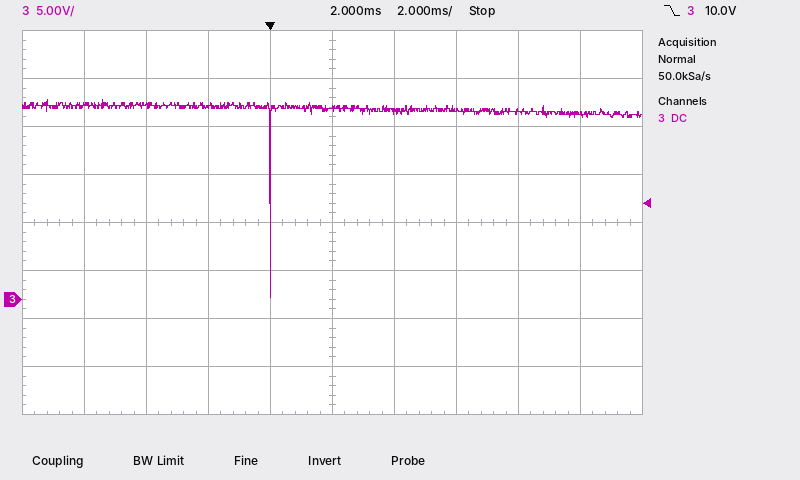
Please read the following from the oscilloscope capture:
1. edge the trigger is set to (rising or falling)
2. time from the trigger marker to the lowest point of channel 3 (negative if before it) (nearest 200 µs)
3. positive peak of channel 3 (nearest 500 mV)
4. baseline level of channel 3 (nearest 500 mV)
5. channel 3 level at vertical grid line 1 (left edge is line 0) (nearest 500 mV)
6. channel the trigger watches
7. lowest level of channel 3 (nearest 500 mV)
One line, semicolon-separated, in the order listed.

falling; 0.0 ms; 21.0 V; 20.0 V; 20.0 V; channel 3; 0.0 V
